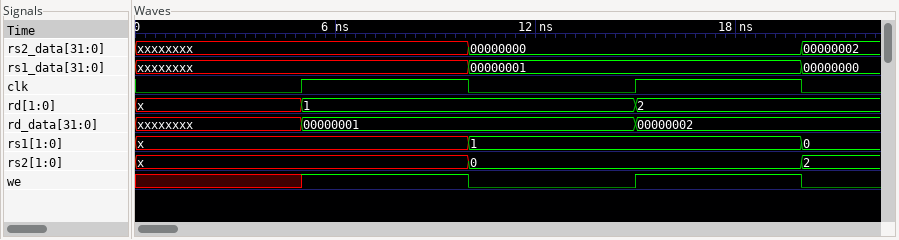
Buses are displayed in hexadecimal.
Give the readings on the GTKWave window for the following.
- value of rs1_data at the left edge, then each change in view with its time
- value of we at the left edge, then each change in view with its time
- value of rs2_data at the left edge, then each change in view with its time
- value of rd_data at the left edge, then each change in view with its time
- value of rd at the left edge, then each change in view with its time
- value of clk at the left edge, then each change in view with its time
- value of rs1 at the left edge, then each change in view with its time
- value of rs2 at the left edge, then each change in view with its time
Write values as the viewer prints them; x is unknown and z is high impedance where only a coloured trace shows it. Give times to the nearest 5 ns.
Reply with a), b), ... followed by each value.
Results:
a) xxxxxxxx, 00000001 at 10 ns, 00000000 at 20 ns
b) x, 1 at 5 ns, 0 at 10 ns, 1 at 15 ns, 0 at 20 ns
c) xxxxxxxx, 00000000 at 10 ns, 00000002 at 20 ns
d) xxxxxxxx, 00000001 at 5 ns, 00000002 at 15 ns
e) x, 1 at 5 ns, 2 at 15 ns
f) 0, 1 at 5 ns, 0 at 10 ns, 1 at 15 ns, 0 at 20 ns
g) x, 1 at 10 ns, 0 at 20 ns
h) x, 0 at 10 ns, 2 at 20 ns
